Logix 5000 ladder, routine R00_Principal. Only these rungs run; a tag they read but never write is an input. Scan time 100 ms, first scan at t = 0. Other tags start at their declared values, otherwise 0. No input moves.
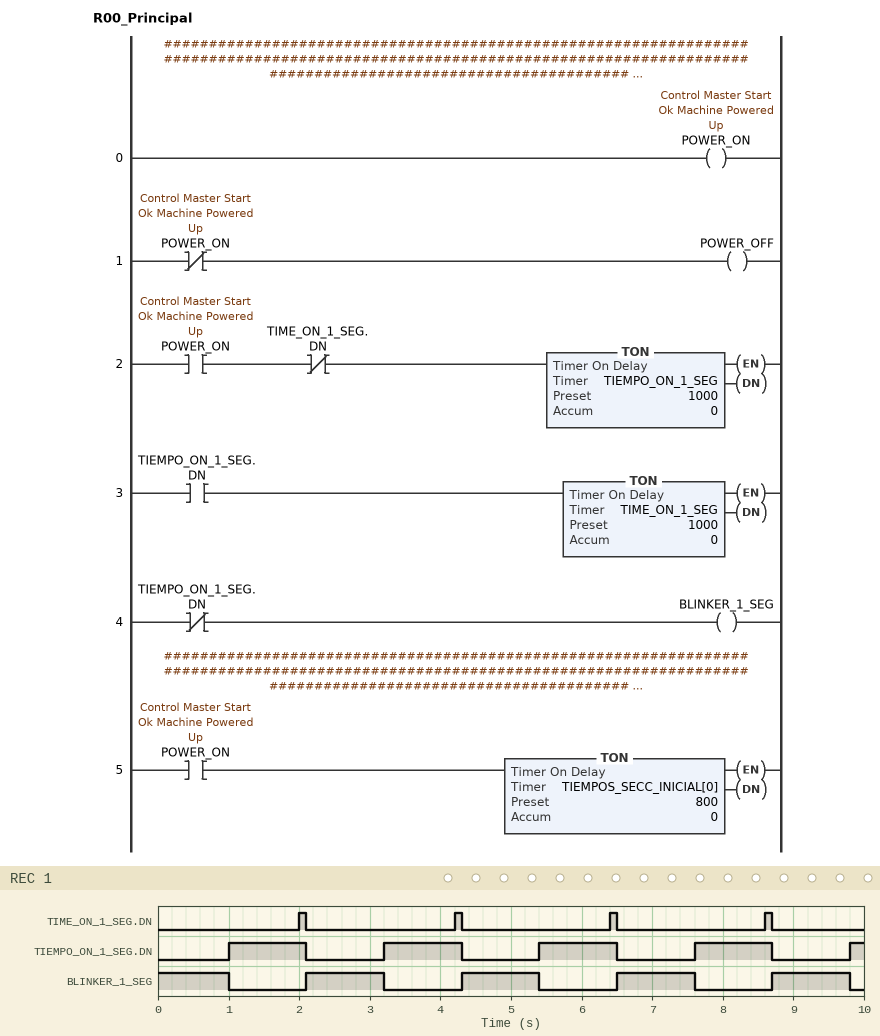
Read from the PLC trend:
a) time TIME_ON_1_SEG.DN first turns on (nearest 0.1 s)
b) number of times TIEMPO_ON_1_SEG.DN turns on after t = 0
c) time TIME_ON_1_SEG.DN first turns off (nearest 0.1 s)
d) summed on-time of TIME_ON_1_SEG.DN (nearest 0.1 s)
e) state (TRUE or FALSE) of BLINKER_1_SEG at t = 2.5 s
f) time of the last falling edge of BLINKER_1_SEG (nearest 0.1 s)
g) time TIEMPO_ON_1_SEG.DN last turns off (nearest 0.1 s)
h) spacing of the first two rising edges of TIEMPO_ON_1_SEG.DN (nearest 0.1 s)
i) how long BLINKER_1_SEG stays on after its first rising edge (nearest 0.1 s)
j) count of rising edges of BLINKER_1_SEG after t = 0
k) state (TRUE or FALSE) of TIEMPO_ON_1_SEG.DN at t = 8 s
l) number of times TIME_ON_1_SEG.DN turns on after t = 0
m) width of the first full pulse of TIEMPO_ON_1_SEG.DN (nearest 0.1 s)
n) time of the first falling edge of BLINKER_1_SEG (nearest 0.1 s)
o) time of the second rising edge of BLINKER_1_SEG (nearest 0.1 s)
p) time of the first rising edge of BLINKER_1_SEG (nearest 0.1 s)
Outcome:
2.0 s
5
2.1 s
0.4 s
TRUE
9.8 s
8.7 s
2.2 s
1.1 s
4
TRUE
4
1.1 s
1.0 s
4.3 s
2.1 s
